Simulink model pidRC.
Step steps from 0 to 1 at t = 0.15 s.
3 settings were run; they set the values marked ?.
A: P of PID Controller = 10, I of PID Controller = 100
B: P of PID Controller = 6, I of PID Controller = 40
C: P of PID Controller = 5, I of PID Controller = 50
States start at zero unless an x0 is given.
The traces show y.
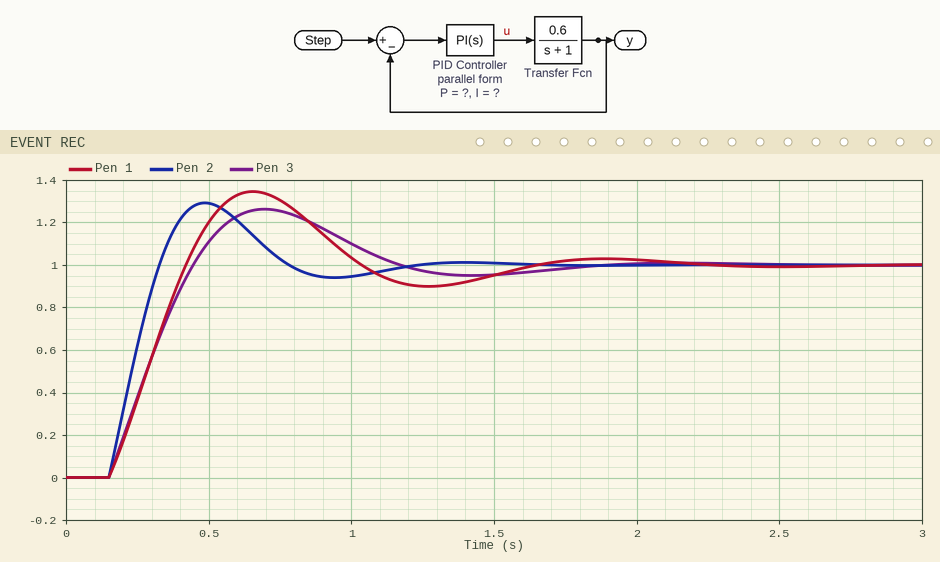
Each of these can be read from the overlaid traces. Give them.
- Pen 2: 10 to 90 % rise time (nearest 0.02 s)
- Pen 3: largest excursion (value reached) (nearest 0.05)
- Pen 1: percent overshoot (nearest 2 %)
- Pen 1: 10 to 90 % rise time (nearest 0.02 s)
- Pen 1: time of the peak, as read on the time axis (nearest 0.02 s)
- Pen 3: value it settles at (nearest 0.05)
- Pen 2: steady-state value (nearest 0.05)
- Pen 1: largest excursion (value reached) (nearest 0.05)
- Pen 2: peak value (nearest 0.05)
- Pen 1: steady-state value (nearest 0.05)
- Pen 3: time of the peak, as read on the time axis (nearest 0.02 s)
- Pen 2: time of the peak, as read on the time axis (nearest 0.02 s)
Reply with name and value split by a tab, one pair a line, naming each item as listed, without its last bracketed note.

Pen 2: 10 to 90 % rise time	0.14 s
Pen 3: largest excursion (value reached)	1.25
Pen 1: percent overshoot	34 %
Pen 1: 10 to 90 % rise time	0.20 s
Pen 1: time of the peak, as read on the time axis	0.66 s
Pen 3: value it settles at	1.00
Pen 2: steady-state value	1.00
Pen 1: largest excursion (value reached)	1.35
Pen 2: peak value	1.30
Pen 1: steady-state value	1.00
Pen 3: time of the peak, as read on the time axis	0.70 s
Pen 2: time of the peak, as read on the time axis	0.48 s
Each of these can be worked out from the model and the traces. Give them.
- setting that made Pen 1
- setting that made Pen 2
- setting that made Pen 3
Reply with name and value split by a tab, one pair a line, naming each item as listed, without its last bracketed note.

setting that made Pen 1	C
setting that made Pen 2	A
setting that made Pen 3	B
